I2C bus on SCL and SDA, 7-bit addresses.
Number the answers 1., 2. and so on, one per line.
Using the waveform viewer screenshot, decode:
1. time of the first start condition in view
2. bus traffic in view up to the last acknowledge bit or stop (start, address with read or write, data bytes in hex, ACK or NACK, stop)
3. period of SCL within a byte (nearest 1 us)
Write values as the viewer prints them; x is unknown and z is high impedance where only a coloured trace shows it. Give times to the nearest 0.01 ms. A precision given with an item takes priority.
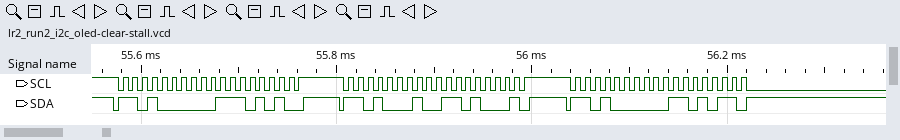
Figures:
1. 55.57 ms
2. start, address 68 write ACK, 75 ACK, stop, start, address 68 read ACK, 68 NACK, stop, start, address 68 write ACK, 6B ACK
3. 10 us
